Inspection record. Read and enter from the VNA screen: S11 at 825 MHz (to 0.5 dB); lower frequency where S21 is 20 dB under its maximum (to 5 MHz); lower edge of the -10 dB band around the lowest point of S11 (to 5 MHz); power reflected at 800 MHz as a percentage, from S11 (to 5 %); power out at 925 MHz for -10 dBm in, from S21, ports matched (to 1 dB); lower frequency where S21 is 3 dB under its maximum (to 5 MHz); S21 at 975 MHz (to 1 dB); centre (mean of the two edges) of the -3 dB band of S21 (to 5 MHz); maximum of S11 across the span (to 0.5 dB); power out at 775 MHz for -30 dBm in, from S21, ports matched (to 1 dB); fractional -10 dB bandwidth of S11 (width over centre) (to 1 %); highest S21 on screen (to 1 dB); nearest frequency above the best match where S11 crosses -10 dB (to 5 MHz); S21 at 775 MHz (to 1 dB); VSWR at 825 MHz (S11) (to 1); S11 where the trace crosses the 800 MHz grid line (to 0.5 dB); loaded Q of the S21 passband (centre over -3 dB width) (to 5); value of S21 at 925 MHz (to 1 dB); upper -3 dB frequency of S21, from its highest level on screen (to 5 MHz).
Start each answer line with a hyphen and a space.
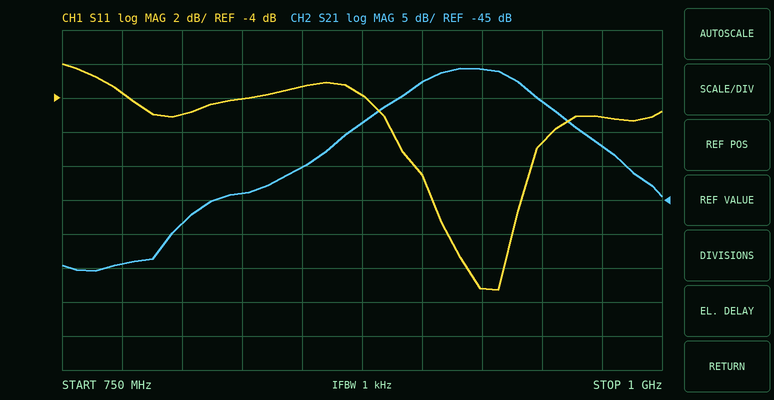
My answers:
- -4.0 dB
- 810 MHz
- 905 MHz
- 30 %
- -36 dBm
- 895 MHz
- -37 dB
- 920 MHz
- -2.0 dB
- -84 dBm
- 4 %
- -26 dB
- 940 MHz
- -54 dB
- 4
- -5.0 dB
- 20
- -26 dB
- 945 MHz
